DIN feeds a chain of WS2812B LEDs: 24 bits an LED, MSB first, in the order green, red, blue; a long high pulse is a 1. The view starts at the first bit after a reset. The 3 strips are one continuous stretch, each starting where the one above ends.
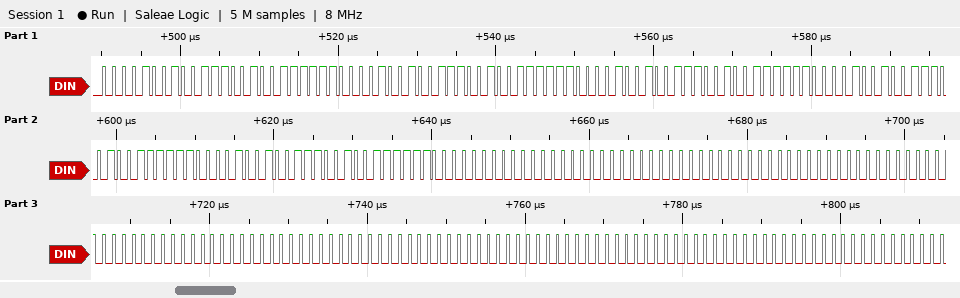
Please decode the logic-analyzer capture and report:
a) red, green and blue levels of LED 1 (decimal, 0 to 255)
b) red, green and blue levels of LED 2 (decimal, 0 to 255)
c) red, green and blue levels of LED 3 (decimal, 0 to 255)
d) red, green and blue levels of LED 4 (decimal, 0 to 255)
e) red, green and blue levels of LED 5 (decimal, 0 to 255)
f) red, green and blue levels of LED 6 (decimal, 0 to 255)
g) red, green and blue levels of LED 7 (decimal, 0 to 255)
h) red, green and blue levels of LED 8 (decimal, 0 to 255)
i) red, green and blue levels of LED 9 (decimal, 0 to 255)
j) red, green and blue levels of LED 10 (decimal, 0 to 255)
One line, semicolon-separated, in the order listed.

57, 9, 63; 57, 9, 63; 57, 9, 63; 57, 9, 63; 57, 9, 63; 0, 0, 0; 0, 0, 0; 0, 0, 0; 0, 0, 0; 0, 0, 0
